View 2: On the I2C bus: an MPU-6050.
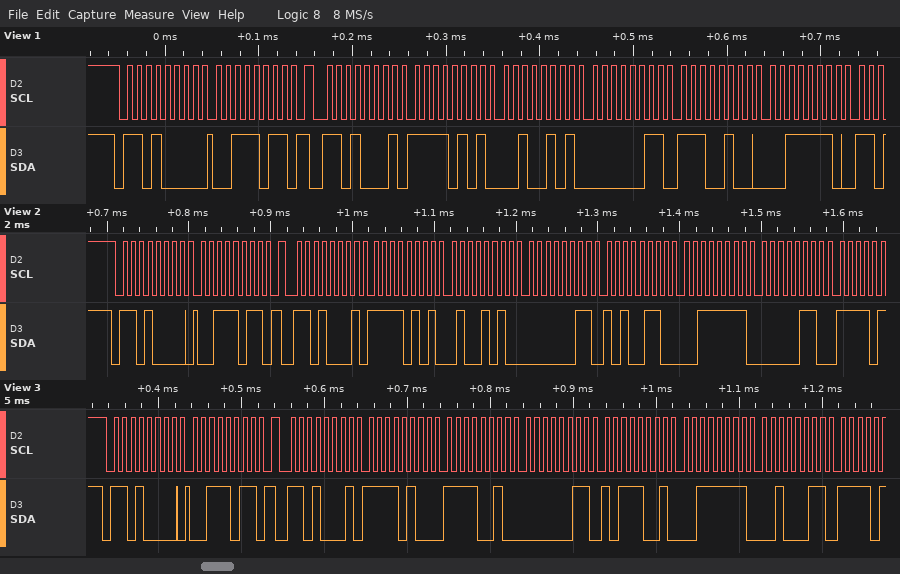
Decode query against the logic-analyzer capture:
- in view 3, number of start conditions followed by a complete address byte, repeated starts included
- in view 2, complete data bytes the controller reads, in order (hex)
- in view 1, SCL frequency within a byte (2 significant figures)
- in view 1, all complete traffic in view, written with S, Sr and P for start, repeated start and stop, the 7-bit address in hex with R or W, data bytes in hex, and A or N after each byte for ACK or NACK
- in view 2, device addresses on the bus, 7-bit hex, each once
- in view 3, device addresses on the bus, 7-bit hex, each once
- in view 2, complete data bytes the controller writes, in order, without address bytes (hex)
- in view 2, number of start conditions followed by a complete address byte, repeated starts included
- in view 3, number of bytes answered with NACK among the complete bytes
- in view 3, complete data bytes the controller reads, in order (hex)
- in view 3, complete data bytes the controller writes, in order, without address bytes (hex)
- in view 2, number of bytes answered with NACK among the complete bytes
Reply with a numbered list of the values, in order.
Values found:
1. 2
2. F5 4A 03 A6 3F 06
3. 100 kHz
4. S 68W A 3B A Sr 68R A F5 A 25 A 03 A E4 A 3E A
5. 0x68
6. 0x68
7. 3B
8. 2
9. 0
10. F4 F2 03 B9 3F 23
11. 3B
12. 0
